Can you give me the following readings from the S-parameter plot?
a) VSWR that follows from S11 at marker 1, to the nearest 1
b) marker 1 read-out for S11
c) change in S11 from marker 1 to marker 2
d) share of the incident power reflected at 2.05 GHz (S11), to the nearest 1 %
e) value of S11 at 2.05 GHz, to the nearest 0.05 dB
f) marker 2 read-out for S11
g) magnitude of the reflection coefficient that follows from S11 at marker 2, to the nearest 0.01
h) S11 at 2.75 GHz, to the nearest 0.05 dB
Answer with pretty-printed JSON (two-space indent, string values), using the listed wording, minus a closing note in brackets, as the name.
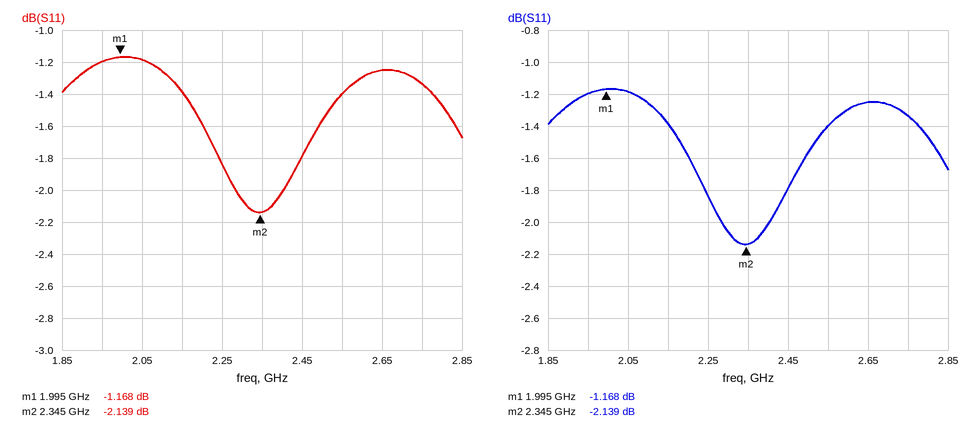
{
  "VSWR that follows from S11 at marker 1, to the nearest 1": "15",
  "marker 1 read-out for S11": "-1.168 dB",
  "change in S11 from marker 1 to marker 2": "-0.971 dB",
  "share of the incident power reflected at 2.05 GHz (S11), to the nearest 1 %": "76 %",
  "value of S11 at 2.05 GHz, to the nearest 0.05 dB": "-1.20 dB",
  "marker 2 read-out for S11": "-2.139 dB",
  "magnitude of the reflection coefficient that follows from S11 at marker 2, to the nearest 0.01": "0.78",
  "S11 at 2.75 GHz, to the nearest 0.05 dB": "-1.35 dB"
}
